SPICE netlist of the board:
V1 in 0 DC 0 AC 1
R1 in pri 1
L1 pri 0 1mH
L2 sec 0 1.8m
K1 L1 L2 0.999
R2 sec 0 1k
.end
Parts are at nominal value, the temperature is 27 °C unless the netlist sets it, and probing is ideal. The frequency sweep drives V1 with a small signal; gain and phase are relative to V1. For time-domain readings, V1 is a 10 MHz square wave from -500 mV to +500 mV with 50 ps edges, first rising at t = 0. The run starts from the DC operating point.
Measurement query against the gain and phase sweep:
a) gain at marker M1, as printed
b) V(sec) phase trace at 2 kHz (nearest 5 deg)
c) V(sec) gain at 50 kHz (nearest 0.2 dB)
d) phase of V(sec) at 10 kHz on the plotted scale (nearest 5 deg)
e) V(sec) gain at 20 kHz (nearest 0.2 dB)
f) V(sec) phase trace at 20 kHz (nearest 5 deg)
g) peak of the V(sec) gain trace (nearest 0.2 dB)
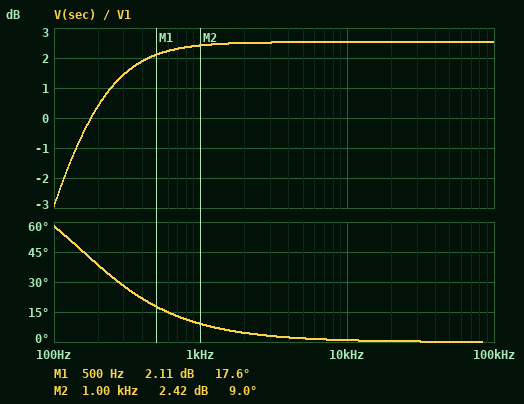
2.11 dB
5 deg
2.6 dB
0 deg
2.6 dB
0 deg
2.6 dB
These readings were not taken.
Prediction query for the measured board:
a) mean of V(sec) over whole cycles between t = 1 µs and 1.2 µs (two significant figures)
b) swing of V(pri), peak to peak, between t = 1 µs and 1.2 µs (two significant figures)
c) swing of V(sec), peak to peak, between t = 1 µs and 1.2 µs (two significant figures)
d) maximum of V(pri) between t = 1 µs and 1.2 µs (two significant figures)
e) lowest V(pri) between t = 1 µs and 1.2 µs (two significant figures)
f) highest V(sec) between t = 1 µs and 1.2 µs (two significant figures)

670 mV
1.0 V
1.3 V
1.0 V
-2.4 mV
1.3 V
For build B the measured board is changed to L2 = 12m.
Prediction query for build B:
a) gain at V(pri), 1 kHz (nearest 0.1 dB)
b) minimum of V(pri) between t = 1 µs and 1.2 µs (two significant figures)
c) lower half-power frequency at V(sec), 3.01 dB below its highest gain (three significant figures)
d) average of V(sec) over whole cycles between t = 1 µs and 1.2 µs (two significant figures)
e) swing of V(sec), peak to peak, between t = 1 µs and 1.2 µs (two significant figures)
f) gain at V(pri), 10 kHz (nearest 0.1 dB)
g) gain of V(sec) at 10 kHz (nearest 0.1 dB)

-0.2 dB
-11 mV
157 Hz
1.7 V
2.7 V
-0.1 dB
10.7 dB
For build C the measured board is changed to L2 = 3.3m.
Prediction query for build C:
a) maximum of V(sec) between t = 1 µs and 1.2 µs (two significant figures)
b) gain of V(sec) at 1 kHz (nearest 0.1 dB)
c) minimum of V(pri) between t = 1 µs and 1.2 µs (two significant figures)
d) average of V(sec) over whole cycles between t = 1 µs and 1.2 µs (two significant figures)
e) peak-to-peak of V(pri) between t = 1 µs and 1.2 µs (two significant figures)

1.8 V
5.0 dB
-3.9 mV
900 mV
1.0 V
